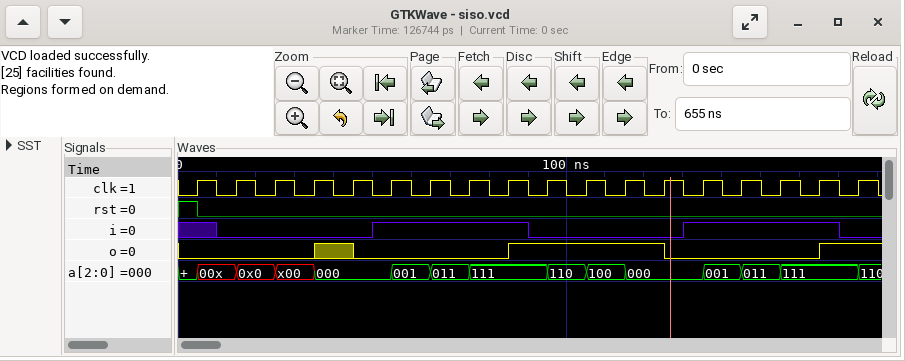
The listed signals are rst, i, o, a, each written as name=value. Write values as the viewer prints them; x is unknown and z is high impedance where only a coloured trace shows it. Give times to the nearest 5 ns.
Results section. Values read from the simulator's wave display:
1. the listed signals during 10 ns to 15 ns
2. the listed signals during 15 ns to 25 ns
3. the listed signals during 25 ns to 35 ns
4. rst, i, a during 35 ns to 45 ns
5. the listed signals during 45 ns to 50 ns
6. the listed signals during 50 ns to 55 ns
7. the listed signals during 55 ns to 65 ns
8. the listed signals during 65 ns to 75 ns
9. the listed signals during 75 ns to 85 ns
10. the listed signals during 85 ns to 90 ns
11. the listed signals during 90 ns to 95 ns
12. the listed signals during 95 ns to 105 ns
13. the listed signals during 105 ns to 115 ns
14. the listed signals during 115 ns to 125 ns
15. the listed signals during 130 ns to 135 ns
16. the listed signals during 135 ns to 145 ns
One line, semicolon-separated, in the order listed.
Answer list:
rst=0, i=0, o=0, a=00x; rst=0, i=0, o=0, a=0x0; rst=0, i=0, o=0, a=x00; rst=0, i=0, a=000; rst=0, i=0, o=0, a=000; rst=0, i=1, o=0, a=000; rst=0, i=1, o=0, a=001; rst=0, i=1, o=0, a=011; rst=0, i=1, o=0, a=111; rst=0, i=1, o=1, a=111; rst=0, i=0, o=1, a=111; rst=0, i=0, o=1, a=110; rst=0, i=0, o=1, a=100; rst=0, i=0, o=1, a=000; rst=0, i=1, o=0, a=000; rst=0, i=1, o=0, a=001
